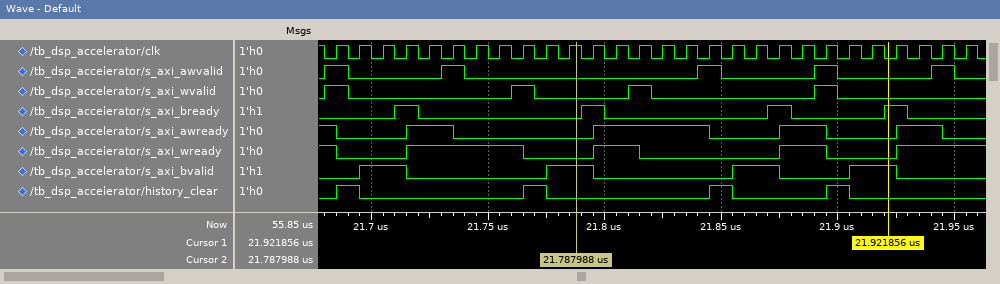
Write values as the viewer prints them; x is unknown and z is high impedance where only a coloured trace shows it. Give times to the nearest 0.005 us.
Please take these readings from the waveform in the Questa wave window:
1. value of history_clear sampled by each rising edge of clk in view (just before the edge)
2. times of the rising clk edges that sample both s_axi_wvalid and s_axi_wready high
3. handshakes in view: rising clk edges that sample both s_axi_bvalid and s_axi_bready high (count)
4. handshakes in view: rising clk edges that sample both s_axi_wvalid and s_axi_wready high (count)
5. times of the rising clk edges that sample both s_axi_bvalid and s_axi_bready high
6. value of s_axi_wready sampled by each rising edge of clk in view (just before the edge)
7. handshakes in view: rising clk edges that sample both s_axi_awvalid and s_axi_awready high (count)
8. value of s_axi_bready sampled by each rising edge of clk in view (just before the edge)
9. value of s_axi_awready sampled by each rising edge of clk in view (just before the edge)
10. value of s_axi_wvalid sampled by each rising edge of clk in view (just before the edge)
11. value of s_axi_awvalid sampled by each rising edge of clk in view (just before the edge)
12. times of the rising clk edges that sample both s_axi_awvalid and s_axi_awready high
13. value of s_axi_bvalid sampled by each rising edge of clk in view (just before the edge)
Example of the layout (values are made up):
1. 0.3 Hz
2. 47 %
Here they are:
1. 0 1 0 0 0 0 0 0 0 1 0 0 0 0 0 0 0 1 0 0 0 0 1 0 0 0 0 0
2. 21.685 us, 21.765 us, 21.815 us, 21.895 us
3. 4
4. 4
5. 21.715 us, 21.795 us, 21.875 us, 21.925 us
6. 1 0 0 0 1 1 1 1 1 0 0 0 1 1 0 0 0 0 0 0 1 1 0 0 0 1 1 1
7. 5
8. 0 0 0 1 0 0 0 0 0 0 0 1 0 0 0 0 0 0 0 1 0 0 0 0 1 0 0 0
9. 1 0 0 0 1 1 0 0 0 0 0 0 1 1 1 1 1 0 0 0 1 1 0 0 0 1 1 0
10. 1 0 0 0 0 0 0 0 1 0 0 0 0 1 0 0 0 0 0 0 0 1 0 0 0 0 0 0
11. 1 0 0 0 0 1 0 0 0 0 0 0 0 0 0 0 1 0 0 0 0 1 0 0 0 0 1 0
12. 21.685 us, 21.735 us, 21.845 us, 21.895 us, 21.945 us
13. 0 0 1 1 0 0 0 0 0 0 1 1 0 0 0 0 0 0 1 1 0 0 0 1 1 0 0 0
